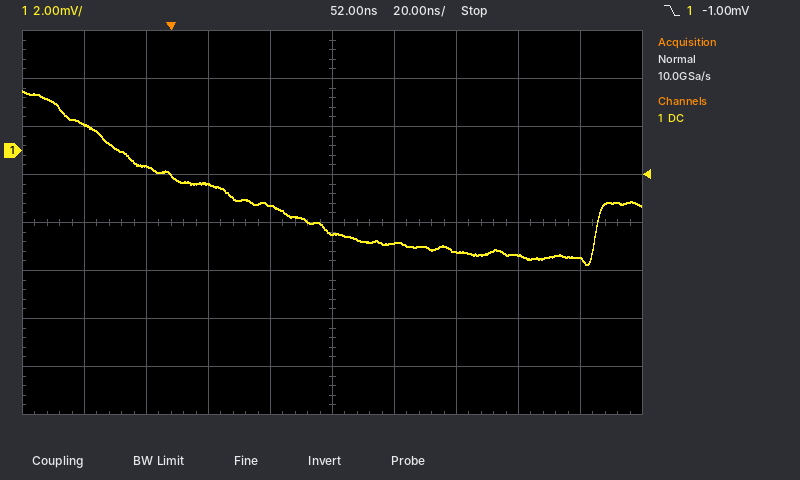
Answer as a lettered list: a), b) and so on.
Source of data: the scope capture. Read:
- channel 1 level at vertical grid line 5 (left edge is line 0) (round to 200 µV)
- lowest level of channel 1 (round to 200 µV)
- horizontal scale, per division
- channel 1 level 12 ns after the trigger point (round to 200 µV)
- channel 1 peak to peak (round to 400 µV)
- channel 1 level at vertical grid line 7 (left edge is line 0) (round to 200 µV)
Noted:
a) -3.4 mV
b) -4.8 mV
c) 20 ns
d) -1.4 mV
e) 7.2 mV
f) -4.2 mV
